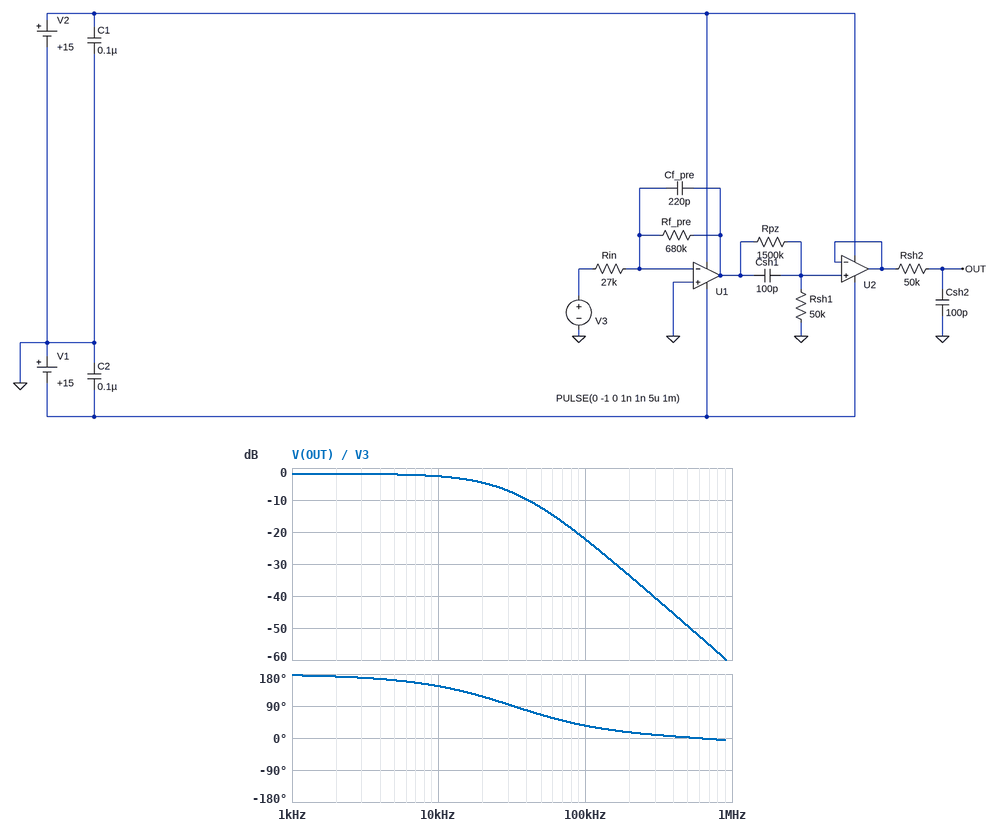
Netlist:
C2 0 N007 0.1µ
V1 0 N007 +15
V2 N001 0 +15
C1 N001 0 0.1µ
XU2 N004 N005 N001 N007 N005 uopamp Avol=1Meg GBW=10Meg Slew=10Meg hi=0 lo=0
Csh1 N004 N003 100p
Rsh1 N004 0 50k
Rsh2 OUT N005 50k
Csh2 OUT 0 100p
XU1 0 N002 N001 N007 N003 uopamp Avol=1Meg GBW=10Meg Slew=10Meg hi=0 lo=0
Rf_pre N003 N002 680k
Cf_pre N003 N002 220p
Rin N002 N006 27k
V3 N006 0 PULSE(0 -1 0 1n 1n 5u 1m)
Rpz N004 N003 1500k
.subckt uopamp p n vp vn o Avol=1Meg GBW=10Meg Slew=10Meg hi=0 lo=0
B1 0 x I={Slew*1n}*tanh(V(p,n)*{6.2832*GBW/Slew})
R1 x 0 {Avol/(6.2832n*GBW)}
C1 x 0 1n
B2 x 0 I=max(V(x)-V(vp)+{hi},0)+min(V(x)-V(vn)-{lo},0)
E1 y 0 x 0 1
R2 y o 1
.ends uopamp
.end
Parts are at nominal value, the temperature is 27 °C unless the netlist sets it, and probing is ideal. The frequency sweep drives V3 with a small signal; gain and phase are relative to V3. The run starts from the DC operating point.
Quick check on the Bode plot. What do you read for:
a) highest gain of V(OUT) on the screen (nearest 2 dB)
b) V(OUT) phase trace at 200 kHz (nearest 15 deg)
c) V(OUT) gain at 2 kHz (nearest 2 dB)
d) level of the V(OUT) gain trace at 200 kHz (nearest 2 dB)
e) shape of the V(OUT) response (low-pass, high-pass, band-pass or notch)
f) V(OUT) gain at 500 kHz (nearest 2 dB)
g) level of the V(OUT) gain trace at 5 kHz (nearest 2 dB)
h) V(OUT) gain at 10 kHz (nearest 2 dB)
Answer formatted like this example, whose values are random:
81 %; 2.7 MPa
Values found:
-2 dB; 15 deg; -2 dB; -34 dB; low-pass; -50 dB; -2 dB; -2 dB
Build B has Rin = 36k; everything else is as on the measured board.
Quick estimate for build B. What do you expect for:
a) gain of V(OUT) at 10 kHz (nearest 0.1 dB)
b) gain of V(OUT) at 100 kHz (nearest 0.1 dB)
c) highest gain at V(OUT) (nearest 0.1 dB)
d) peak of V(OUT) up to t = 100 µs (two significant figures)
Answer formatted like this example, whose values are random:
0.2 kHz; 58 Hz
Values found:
-5.1 dB; -24.8 dB; -4.3 dB; 220 mV
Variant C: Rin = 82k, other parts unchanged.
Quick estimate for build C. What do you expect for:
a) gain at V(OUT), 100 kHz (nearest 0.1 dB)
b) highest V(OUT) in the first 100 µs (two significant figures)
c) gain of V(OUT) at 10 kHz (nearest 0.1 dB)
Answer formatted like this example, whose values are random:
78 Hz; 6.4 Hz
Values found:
-31.9 dB; 96 mV; -12.2 dB
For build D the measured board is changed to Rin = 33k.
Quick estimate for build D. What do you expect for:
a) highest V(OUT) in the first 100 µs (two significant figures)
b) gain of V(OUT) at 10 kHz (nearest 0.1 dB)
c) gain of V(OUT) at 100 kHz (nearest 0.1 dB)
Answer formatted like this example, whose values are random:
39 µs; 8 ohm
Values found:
240 mV; -4.3 dB; -24.0 dB
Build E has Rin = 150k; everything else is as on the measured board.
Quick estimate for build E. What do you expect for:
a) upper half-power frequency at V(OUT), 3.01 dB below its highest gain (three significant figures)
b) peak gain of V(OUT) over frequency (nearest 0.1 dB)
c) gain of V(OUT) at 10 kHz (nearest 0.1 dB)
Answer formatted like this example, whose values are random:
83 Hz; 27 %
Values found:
20.9 kHz; -16.7 dB; -17.5 dB
